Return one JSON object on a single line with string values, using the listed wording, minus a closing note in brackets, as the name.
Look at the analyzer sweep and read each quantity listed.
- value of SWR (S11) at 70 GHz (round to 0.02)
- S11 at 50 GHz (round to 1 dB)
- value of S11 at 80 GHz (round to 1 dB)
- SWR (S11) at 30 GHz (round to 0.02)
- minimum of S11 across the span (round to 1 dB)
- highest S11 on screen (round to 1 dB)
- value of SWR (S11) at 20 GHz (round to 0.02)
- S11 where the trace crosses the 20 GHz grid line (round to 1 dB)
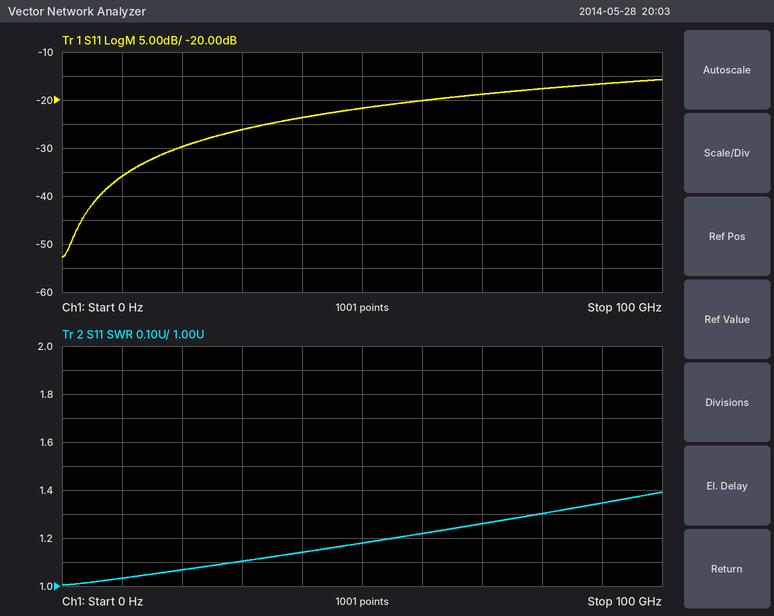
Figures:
{"value of SWR (S11) at 70 GHz": "1.26", "S11 at 50 GHz": "-22 dB", "value of S11 at 80 GHz": "-18 dB", "SWR (S11) at 30 GHz": "1.10", "minimum of S11 across the span": "-53 dB", "highest S11 on screen": "-16 dB", "value of SWR (S11) at 20 GHz": "1.06", "S11 where the trace crosses the 20 GHz grid line": "-30 dB"}
